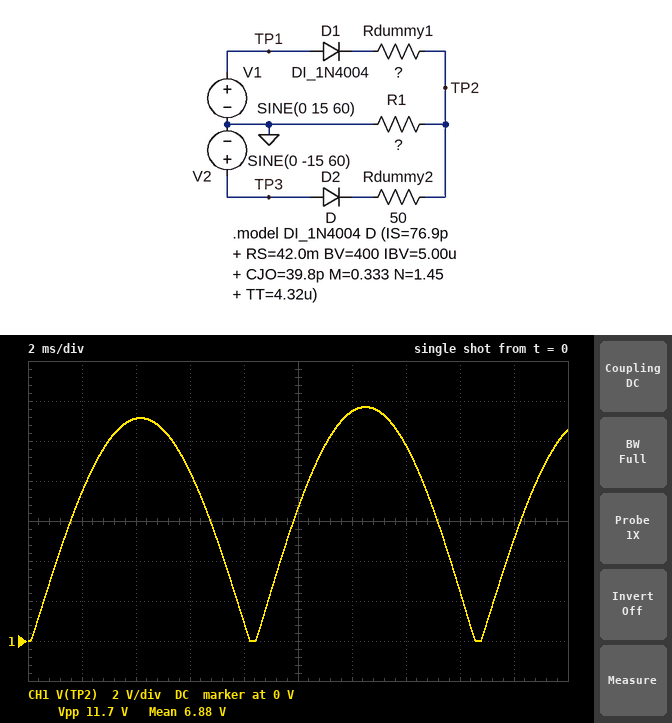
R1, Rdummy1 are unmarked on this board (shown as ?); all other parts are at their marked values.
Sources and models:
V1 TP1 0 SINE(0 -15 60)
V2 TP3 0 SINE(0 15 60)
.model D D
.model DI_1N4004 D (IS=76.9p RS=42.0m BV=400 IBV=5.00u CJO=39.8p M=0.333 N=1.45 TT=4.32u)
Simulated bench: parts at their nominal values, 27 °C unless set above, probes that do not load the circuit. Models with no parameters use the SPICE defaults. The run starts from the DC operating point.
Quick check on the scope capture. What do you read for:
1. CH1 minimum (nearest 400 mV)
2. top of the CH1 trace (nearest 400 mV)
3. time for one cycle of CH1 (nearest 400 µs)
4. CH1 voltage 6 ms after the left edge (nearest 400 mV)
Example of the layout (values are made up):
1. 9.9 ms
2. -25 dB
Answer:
1. 0 V
2. 11.6 V
3. 8.4 ms
4. 8.4 V
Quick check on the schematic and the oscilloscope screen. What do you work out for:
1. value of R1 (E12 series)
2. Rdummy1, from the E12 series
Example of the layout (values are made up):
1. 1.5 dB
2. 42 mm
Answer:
1. 180 Ω
2. 39 Ω
